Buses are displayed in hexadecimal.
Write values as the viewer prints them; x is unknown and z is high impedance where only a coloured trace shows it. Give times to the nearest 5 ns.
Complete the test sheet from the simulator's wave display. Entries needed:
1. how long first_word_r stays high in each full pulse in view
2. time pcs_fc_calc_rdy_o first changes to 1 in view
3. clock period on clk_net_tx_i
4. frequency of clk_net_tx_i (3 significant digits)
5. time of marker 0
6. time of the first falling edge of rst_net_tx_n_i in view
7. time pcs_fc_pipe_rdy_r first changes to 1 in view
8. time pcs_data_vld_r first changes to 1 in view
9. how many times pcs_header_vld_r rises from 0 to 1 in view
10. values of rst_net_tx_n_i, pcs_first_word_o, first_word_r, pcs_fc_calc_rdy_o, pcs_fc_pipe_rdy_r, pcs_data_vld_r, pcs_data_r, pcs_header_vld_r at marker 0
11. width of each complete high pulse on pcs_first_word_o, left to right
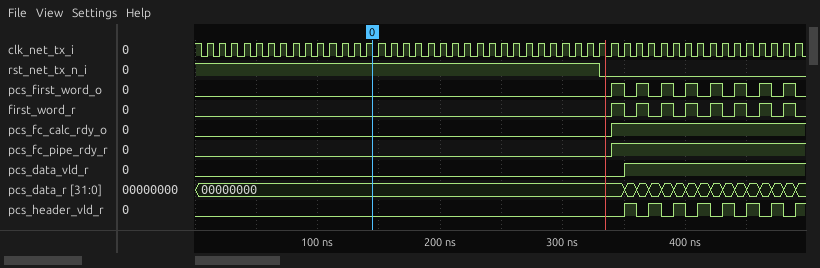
10 ns, 10 ns, 10 ns, 10 ns, 10 ns, 10 ns, 10 ns, 10 ns
340 ns
10 ns
100 MHz
145 ns
330 ns
340 ns
350 ns
8
rst_net_tx_n_i=1, pcs_first_word_o=0, first_word_r=0, pcs_fc_calc_rdy_o=0, pcs_fc_pipe_rdy_r=0, pcs_data_vld_r=0, pcs_data_r=00000000, pcs_header_vld_r=0
10 ns, 10 ns, 10 ns, 10 ns, 10 ns, 10 ns, 10 ns, 10 ns
